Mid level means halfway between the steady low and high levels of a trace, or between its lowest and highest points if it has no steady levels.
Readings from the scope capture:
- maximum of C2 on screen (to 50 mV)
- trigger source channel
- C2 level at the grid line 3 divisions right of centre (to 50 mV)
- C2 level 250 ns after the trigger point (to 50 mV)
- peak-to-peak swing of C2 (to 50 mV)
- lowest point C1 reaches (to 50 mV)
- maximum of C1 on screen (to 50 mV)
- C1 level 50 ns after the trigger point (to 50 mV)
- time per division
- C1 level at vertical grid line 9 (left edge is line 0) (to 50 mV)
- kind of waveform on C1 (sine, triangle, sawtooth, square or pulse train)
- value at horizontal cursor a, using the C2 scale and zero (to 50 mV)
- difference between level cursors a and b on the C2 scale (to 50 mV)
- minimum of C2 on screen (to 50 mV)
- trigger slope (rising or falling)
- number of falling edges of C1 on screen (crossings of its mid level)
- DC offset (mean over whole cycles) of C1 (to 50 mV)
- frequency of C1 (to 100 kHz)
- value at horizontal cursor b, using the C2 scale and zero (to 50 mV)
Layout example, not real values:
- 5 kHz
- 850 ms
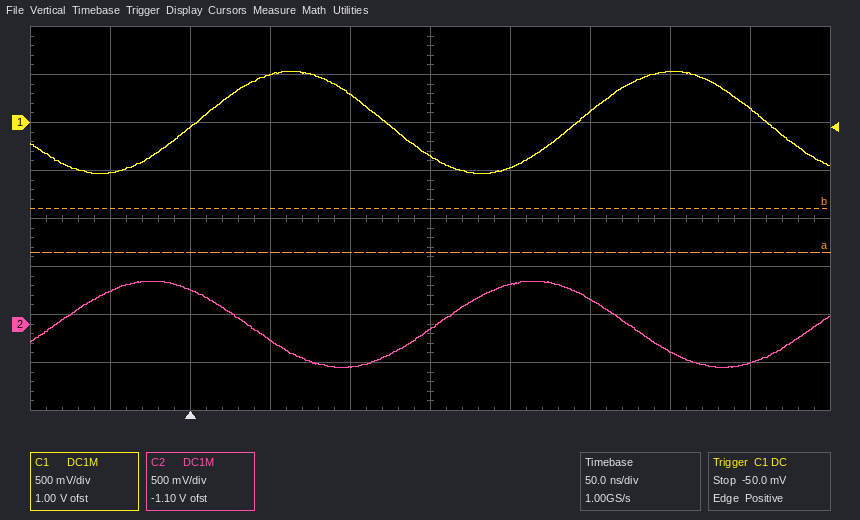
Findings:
- 450 mV
- C1
- -300 mV
- 250 mV
- 900 mV
- -550 mV
- 550 mV
- 500 mV
- 50 ns
- 150 mV
- sine
- 750 mV
- 450 mV
- -450 mV
- rising
- 2
- 0 mV
- 4.2 MHz
- 1.20 V
